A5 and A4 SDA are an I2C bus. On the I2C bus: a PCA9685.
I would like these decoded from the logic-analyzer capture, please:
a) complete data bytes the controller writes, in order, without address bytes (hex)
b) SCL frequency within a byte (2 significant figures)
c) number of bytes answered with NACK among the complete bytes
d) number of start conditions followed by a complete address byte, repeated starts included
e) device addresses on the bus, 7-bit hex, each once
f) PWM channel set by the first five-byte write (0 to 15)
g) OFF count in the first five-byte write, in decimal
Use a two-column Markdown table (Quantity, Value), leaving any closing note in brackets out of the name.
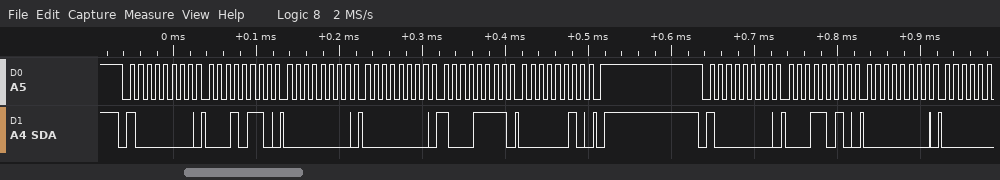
| Quantity | Value |
|---|---|
| complete data bytes the controller writes, in order, without address bytes | 16 00 00 8F 02 1A 00 |
| SCL frequency within a byte | 100 kHz |
| number of bytes answered with NACK among the complete bytes | 0 |
| number of start conditions followed by a complete address byte, repeated starts included | 2 |
| device addresses on the bus, 7-bit hex, each once | 0x40 |
| PWM channel set by the first five-byte write | 4 |
| OFF count in the first five-byte write, in decimal | 655 |
